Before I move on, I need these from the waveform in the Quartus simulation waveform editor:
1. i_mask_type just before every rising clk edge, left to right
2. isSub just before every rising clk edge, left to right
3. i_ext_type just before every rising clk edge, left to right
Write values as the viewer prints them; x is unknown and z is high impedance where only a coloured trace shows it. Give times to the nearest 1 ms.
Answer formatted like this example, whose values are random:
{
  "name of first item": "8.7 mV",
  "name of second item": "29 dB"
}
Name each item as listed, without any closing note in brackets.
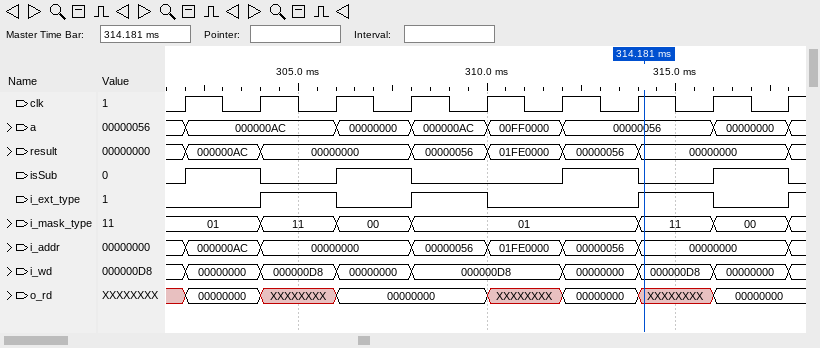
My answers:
{
  "i_mask_type just before every rising clk edge, left to right": "01, 01, 11, 00, 01, 01, 01, 11, 00",
  "isSub just before every rising clk edge, left to right": "0 1 0 1 0 0 1 0 1",
  "i_ext_type just before every rising clk edge, left to right": "0 0 1 0 1 0 0 1 0"
}
